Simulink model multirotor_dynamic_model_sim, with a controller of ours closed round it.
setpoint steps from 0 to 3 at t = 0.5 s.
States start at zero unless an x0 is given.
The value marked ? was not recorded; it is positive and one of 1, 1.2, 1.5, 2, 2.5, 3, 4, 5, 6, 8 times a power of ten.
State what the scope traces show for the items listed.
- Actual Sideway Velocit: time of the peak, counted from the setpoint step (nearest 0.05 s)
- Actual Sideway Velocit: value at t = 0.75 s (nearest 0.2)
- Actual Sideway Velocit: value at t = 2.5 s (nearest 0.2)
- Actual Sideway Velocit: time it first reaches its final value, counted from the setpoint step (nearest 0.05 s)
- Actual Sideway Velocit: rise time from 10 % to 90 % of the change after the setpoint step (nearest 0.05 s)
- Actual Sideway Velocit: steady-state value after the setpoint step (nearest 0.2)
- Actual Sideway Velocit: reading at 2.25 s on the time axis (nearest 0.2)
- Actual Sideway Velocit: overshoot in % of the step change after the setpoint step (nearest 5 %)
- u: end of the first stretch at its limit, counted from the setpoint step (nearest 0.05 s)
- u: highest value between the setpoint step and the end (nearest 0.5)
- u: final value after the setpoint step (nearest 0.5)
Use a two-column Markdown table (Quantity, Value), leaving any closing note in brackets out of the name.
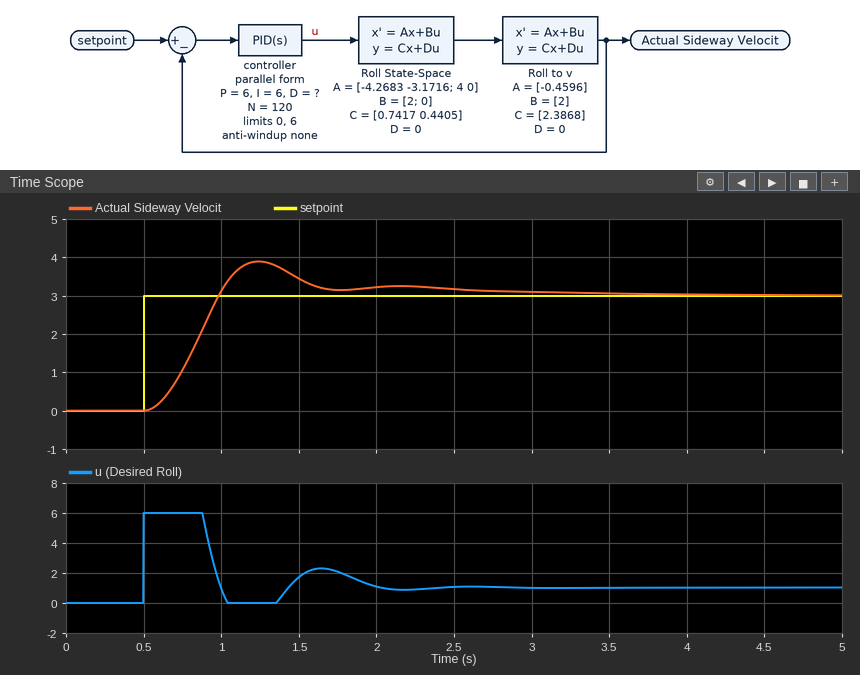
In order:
| Quantity | Value |
|---|---|
| Actual Sideway Velocit: time of the peak, counted from the setpoint step | 0.75 s |
| Actual Sideway Velocit: value at t = 0.75 s | 1.0 |
| Actual Sideway Velocit: value at t = 2.5 s | 3.2 |
| Actual Sideway Velocit: time it first reaches its final value, counted from the setpoint step | 0.50 s |
| Actual Sideway Velocit: rise time from 10 % to 90 % of the change after the setpoint step | 0.30 s |
| Actual Sideway Velocit: steady-state value after the setpoint step | 3.0 |
| Actual Sideway Velocit: reading at 2.25 s on the time axis | 3.2 |
| Actual Sideway Velocit: overshoot in % of the step change after the setpoint step | 30 % |
| u: end of the first stretch at its limit, counted from the setpoint step | 0.40 s |
| u: highest value between the setpoint step and the end | 6.0 |
| u: final value after the setpoint step | 1.0 |
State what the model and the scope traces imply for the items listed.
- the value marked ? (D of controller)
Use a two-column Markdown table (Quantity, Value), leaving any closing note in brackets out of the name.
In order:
| Quantity | Value |
|---|---|
| the value marked ? | 0.5 |
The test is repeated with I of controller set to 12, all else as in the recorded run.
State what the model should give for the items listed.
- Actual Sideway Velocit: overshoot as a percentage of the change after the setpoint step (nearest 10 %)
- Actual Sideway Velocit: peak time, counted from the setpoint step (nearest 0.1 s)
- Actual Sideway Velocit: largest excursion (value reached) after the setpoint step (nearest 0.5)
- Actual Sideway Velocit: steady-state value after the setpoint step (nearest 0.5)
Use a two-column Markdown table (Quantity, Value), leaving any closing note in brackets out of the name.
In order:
| Quantity | Value |
|---|---|
| Actual Sideway Velocit: overshoot as a percentage of the change after the setpoint step | 50 % |
| Actual Sideway Velocit: peak time, counted from the setpoint step | 0.8 s |
| Actual Sideway Velocit: largest excursion (value reached) after the setpoint step | 4.5 |
| Actual Sideway Velocit: steady-state value after the setpoint step | 3.0 |
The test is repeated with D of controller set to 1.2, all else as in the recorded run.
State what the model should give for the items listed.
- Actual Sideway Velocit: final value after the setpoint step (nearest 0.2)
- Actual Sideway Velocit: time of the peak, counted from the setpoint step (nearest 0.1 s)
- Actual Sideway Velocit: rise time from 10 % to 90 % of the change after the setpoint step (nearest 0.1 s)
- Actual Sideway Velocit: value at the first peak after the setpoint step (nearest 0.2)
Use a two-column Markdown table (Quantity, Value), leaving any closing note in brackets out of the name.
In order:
| Quantity | Value |
|---|---|
| Actual Sideway Velocit: final value after the setpoint step | 3.0 |
| Actual Sideway Velocit: time of the peak, counted from the setpoint step | 1.0 s |
| Actual Sideway Velocit: rise time from 10 % to 90 % of the change after the setpoint step | 0.4 s |
| Actual Sideway Velocit: value at the first peak after the setpoint step | 3.4 |
